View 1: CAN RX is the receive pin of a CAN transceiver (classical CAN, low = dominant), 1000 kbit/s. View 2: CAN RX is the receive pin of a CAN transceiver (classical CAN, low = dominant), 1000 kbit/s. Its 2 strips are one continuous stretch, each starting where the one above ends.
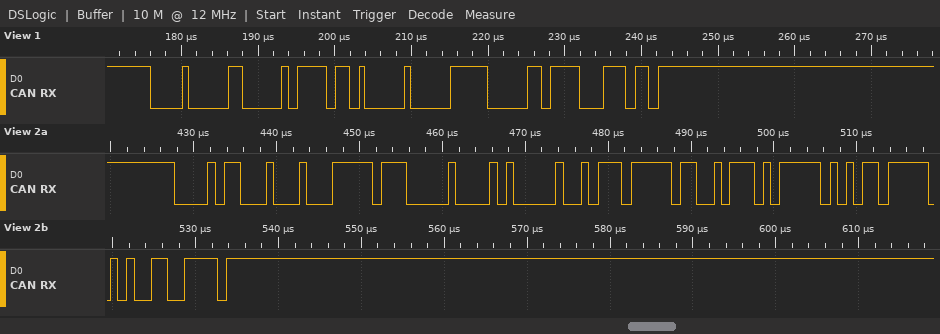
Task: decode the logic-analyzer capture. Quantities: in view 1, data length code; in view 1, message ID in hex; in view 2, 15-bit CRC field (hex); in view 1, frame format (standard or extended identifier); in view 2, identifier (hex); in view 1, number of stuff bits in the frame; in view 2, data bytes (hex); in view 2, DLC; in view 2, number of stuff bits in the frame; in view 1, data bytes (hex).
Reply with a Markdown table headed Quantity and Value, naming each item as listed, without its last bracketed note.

| Quantity | Value |
|---|---|
| in view 1, data length code | 3 |
| in view 1, message ID in hex | 0x082 |
| in view 2, 15-bit CRC field | 0x7A67 |
| in view 1, frame format | standard |
| in view 2, identifier | 0x0B1 |
| in view 1, number of stuff bits in the frame | 6 |
| in view 2, data bytes | FF 00 50 17 7F 2E BF 5B |
| in view 2, DLC | 8 |
| in view 2, number of stuff bits in the frame | 6 |
| in view 1, data bytes | DA 00 78 |
